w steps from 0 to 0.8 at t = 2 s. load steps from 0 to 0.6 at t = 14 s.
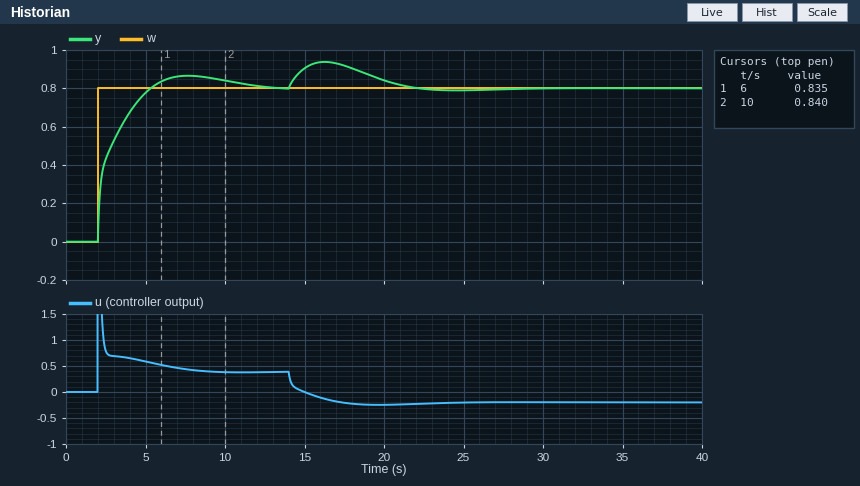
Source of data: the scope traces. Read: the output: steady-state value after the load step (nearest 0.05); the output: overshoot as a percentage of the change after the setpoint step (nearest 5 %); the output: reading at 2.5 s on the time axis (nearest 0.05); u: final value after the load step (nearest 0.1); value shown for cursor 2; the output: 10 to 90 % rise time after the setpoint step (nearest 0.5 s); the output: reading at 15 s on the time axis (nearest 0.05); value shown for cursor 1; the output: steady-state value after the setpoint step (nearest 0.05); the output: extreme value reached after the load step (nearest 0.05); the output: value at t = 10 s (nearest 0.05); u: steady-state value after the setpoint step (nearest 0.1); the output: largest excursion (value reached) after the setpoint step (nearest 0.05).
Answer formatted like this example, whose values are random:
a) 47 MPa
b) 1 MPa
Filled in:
a) 0.80
b) 10 %
c) 0.45
d) -0.2
e) 0.840
f) 2.5 s
g) 0.90
h) 0.835
i) 0.80
j) 0.95
k) 0.85
l) 0.4
m) 0.85
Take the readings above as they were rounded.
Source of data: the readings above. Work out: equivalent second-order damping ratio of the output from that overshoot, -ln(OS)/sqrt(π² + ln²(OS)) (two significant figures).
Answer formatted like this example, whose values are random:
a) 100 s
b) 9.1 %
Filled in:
a) 0.59
